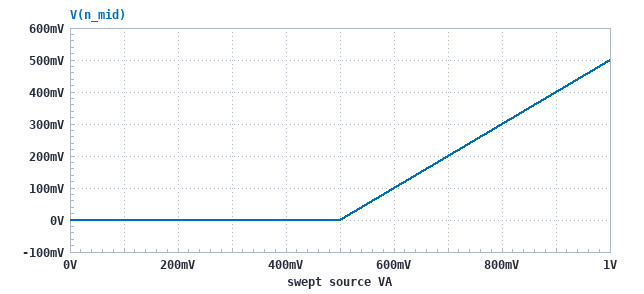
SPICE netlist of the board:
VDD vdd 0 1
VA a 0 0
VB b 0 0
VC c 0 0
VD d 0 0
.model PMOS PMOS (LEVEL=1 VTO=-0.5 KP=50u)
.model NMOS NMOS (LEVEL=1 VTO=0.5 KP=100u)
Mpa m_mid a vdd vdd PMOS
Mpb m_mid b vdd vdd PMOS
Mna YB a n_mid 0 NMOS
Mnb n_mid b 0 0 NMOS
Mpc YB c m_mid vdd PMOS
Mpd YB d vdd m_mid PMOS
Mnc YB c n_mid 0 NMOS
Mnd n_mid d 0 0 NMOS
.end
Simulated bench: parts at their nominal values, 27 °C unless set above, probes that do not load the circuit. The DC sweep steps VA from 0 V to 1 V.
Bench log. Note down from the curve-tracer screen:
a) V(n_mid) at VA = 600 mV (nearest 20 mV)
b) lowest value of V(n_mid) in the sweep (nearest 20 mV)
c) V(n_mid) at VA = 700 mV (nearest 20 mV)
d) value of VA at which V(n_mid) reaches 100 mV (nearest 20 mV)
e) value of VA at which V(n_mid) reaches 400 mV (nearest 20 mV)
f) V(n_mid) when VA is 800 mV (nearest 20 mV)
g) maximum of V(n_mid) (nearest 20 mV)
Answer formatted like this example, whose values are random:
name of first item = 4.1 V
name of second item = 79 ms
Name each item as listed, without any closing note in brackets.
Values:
V(n_mid) at VA = 600 mV = 100 mV
lowest value of V(n_mid) in the sweep = 0 V
V(n_mid) at VA = 700 mV = 200 mV
value of VA at which V(n_mid) reaches 100 mV = 600 mV
value of VA at which V(n_mid) reaches 400 mV = 900 mV
V(n_mid) when VA is 800 mV = 300 mV
maximum of V(n_mid) = 500 mV
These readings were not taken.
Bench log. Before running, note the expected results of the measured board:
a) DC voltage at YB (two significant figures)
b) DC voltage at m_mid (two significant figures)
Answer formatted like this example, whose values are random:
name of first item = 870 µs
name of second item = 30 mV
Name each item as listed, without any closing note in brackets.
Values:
DC voltage at YB = 1.0 V
DC voltage at m_mid = 1.0 V
